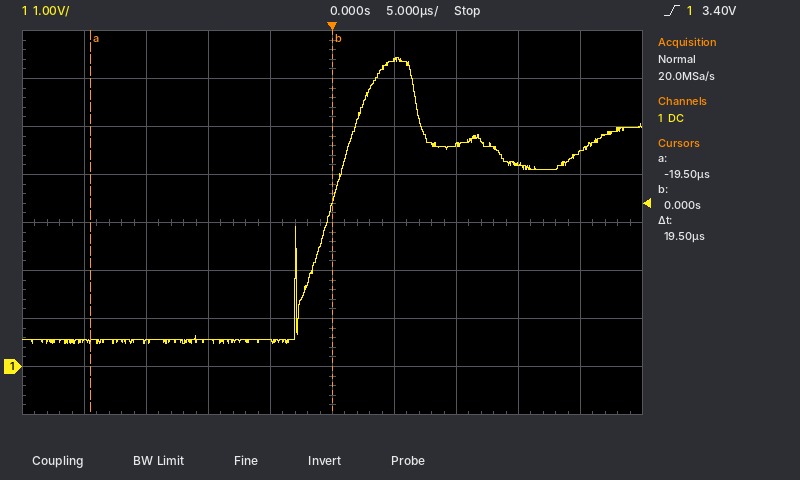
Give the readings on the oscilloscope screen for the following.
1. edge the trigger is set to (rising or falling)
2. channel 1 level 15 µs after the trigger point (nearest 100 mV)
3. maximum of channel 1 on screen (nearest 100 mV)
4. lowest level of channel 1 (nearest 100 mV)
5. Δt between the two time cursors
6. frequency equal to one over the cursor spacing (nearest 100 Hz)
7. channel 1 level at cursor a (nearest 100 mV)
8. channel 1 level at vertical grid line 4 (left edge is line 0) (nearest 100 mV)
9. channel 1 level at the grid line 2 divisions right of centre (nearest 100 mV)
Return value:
rising
4.2 V
6.4 V
500 mV
19.5 µs
51.3 kHz
500 mV
500 mV
4.6 V
